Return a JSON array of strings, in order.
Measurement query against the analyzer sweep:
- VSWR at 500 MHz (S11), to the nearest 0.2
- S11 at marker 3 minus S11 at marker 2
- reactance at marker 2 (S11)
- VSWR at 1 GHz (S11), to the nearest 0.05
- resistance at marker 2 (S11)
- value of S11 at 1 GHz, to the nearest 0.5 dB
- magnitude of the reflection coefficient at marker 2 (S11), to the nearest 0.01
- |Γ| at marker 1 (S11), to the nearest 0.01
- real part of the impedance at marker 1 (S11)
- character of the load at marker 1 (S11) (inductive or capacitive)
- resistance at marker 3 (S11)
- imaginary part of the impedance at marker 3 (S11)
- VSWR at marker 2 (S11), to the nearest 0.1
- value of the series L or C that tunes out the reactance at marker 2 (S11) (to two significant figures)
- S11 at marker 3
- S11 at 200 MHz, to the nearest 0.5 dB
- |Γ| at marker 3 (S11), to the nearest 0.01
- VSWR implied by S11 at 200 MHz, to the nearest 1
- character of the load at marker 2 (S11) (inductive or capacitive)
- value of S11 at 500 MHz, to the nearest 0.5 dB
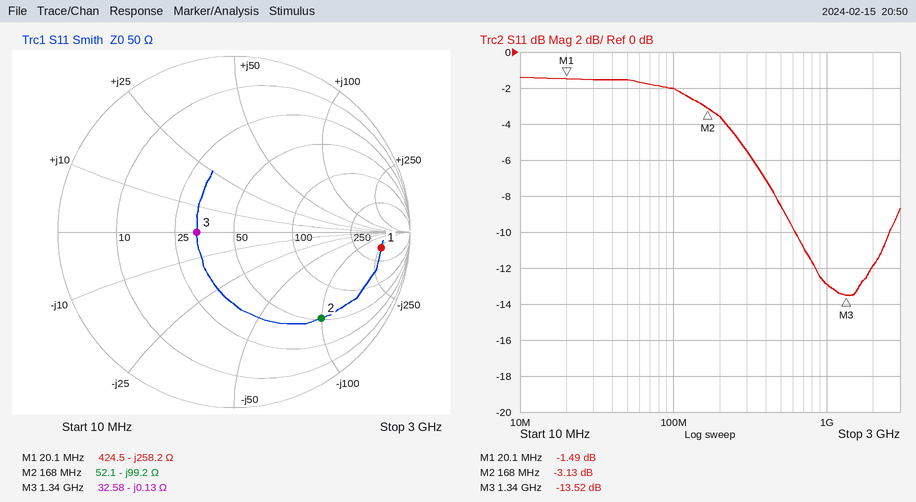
["2.2", "-10.39 dB", "-99.2 Ω", "1.60", "52.1 Ω", "-13.0 dB", "0.70", "0.84", "424.5 Ω", "capacitive", "32.58 Ω", "-0.13 Ω", "5.6", "94 nH", "-13.52 dB", "-3.5 dB", "0.21", "5", "capacitive", "-8.5 dB"]
